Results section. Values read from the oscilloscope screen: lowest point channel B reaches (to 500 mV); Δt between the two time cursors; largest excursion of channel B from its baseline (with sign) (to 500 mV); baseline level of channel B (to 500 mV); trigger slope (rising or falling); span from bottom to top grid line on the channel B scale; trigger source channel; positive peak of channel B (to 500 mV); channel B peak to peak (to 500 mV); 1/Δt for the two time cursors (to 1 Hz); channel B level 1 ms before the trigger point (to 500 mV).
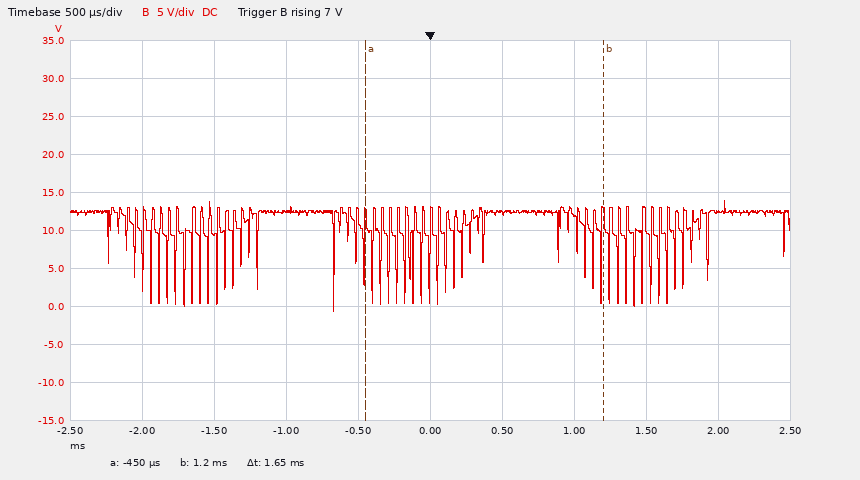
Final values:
-500 mV
1.65 ms
-13.0 V
12.5 V
rising
50 V
channel B
14.0 V
14.5 V
606 Hz
12.5 V
